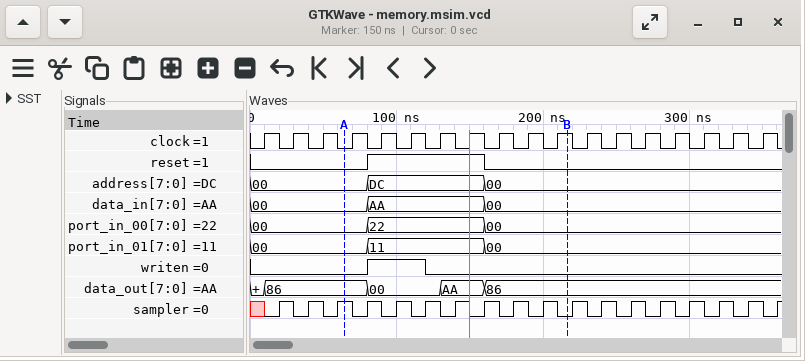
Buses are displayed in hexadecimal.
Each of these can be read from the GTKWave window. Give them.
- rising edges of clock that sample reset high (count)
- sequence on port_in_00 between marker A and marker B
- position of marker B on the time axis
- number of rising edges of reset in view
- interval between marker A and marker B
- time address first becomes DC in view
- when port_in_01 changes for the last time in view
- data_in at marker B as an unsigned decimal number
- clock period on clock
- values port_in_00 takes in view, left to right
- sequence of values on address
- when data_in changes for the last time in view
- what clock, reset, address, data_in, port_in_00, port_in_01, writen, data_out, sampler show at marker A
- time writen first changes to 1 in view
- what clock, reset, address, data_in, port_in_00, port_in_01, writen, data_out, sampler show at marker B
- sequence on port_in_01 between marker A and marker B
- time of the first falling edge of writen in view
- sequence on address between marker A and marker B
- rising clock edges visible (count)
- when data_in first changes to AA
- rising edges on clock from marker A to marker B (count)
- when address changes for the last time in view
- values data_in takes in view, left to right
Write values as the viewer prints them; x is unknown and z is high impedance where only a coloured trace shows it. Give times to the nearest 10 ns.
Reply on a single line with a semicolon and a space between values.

4; 00, 22, 00; 220 ns; 1; 150 ns; 80 ns; 160 ns; 0; 20 ns; 00, 22, 00; 00, DC, 00; 160 ns; clock=0, reset=0, address=00, data_in=00, port_in_00=00, port_in_01=00, writen=0, data_out=86, sampler=1; 80 ns; clock=1, reset=0, address=00, data_in=00, port_in_00=00, port_in_01=00, writen=0, data_out=86, sampler=0; 00, 11, 00; 120 ns; 00, DC, 00; 18; 80 ns; 8; 160 ns; 00, AA, 00
